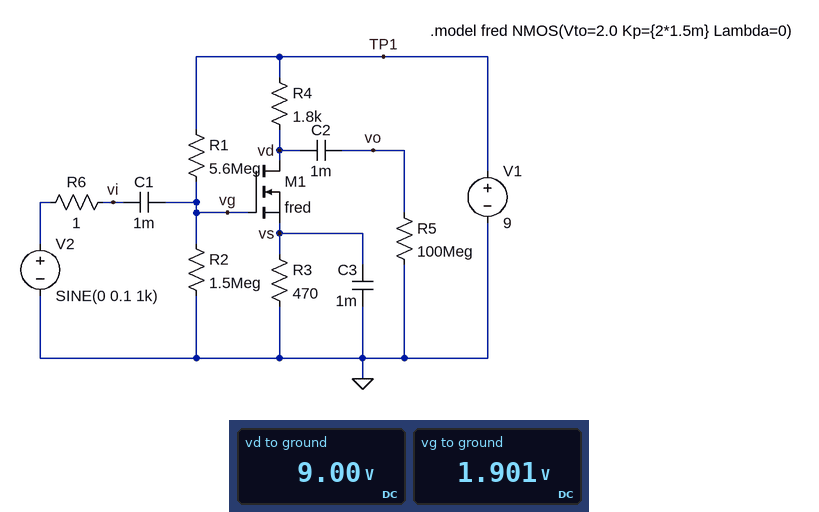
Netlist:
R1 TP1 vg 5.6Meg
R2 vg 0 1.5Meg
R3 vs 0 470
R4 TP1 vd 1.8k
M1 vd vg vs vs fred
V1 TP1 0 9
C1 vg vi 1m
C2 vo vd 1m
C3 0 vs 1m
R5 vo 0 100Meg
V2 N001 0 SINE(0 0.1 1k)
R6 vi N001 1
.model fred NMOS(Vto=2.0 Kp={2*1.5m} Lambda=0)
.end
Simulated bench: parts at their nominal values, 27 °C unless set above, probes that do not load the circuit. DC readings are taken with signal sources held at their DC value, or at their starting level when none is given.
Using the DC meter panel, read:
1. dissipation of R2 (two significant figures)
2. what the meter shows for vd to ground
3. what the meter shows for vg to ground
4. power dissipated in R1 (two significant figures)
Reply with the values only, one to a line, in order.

2.4 µW
9.00 V
1.901 V
9.0 µW
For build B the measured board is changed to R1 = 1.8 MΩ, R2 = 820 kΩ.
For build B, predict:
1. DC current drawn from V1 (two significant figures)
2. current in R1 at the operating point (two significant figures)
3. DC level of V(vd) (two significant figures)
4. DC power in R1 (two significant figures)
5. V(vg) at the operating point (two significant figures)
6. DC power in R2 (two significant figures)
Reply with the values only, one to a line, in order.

510 µA
3.4 µA
8.1 V
21 µW
2.8 V
9.7 µW
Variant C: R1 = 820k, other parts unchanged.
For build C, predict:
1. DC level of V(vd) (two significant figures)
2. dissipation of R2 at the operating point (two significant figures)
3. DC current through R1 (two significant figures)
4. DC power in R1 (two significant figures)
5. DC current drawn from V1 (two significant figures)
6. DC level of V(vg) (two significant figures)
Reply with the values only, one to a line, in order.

2.4 V
23 µW
3.9 µA
12 µW
3.7 mA
5.8 V
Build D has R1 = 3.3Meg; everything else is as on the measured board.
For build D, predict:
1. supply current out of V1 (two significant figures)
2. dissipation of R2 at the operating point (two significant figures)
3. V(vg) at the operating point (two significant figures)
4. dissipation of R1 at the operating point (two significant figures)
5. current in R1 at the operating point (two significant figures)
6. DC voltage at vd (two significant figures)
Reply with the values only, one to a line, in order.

500 µA
5.3 µW
2.8 V
12 µW
1.9 µA
8.1 V
